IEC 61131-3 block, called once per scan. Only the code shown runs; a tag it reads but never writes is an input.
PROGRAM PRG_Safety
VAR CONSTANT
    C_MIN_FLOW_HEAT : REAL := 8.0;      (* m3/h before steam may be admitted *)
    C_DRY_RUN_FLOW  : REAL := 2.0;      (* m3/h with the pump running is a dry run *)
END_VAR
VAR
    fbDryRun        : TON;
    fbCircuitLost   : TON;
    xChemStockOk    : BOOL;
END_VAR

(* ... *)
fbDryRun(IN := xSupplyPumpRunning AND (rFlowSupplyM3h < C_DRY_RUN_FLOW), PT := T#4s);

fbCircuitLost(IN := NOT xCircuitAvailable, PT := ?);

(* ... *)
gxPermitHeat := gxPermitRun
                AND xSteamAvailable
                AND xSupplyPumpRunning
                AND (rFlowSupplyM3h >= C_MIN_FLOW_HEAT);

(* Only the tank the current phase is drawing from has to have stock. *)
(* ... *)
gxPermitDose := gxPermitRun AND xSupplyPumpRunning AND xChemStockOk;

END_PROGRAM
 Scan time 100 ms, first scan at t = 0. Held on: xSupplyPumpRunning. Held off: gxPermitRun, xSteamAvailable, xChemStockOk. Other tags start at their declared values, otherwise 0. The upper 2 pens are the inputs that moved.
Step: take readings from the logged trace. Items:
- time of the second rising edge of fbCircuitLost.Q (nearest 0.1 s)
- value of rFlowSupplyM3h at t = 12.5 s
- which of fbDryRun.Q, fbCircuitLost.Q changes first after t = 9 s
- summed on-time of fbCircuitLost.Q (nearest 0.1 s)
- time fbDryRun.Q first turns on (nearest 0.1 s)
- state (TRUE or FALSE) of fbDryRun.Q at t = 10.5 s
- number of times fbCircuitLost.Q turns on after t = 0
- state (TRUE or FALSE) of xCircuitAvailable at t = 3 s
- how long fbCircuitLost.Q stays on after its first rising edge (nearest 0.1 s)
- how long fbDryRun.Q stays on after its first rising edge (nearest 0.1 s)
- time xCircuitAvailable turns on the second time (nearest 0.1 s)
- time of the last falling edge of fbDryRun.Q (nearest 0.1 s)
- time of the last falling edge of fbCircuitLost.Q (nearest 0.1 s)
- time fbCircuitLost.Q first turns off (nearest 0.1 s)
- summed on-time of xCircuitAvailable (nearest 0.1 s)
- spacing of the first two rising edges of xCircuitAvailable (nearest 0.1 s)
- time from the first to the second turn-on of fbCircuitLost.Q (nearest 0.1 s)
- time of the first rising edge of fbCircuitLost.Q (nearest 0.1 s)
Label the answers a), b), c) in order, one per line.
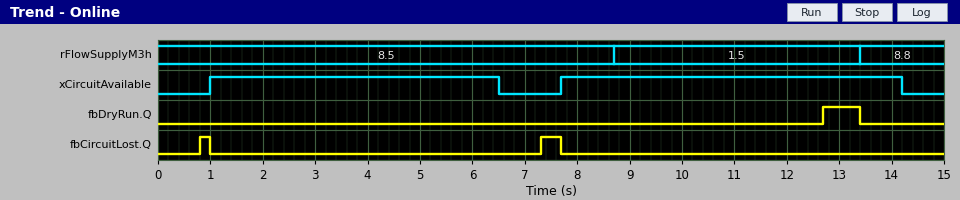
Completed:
a) 7.3 s
b) 1.5
c) fbDryRun.Q
d) 0.6 s
e) 12.7 s
f) FALSE
g) 2
h) TRUE
i) 0.2 s
j) 0.7 s
k) 7.7 s
l) 13.4 s
m) 7.7 s
n) 1.0 s
o) 12.0 s
p) 6.7 s
q) 6.5 s
r) 0.8 s
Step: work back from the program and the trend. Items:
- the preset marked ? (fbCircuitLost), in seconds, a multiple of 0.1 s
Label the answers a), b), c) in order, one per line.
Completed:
a) 0.8 s
